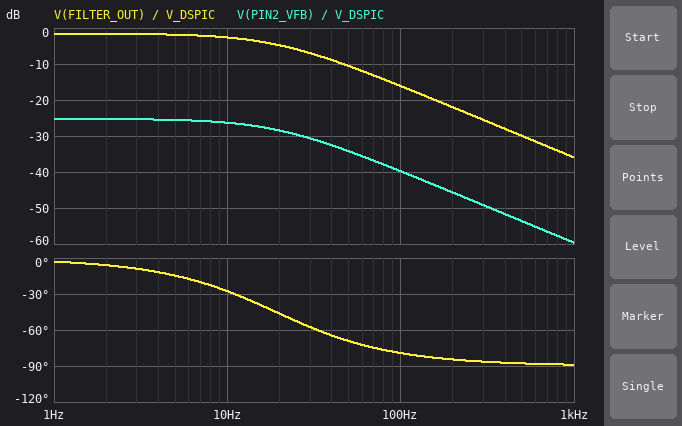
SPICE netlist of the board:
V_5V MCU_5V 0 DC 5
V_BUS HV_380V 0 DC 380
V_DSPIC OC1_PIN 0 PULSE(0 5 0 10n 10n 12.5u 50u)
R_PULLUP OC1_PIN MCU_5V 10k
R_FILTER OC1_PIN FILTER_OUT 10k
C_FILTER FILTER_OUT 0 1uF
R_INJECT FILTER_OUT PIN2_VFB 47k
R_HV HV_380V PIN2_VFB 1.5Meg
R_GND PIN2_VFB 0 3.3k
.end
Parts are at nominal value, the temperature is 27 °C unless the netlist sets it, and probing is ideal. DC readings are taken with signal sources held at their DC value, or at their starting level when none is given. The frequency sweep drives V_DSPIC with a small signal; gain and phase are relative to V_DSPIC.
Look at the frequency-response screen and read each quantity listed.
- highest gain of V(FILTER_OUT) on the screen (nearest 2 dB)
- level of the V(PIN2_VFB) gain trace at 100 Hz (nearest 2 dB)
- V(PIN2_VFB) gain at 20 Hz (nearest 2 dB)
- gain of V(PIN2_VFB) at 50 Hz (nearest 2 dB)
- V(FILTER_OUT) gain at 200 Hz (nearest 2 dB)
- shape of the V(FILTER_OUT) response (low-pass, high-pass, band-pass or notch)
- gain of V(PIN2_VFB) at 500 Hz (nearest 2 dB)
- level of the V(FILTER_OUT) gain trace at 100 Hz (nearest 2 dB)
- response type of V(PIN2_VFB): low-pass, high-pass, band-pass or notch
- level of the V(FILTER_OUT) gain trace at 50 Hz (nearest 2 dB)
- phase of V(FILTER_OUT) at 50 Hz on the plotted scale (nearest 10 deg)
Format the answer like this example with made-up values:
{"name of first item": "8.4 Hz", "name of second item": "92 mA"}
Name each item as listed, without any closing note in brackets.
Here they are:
{"highest gain of V(FILTER_OUT) on the screen": "-2 dB", "level of the V(PIN2_VFB) gain trace at 100 Hz": "-40 dB", "V(PIN2_VFB) gain at 20 Hz": "-28 dB", "gain of V(PIN2_VFB) at 50 Hz": "-34 dB", "V(FILTER_OUT) gain at 200 Hz": "-22 dB", "shape of the V(FILTER_OUT) response": "low-pass", "gain of V(PIN2_VFB) at 500 Hz": "-54 dB", "level of the V(FILTER_OUT) gain trace at 100 Hz": "-16 dB", "response type of V(PIN2_VFB): low-pass, high-pass, band-pass or notch": "low-pass", "level of the V(FILTER_OUT) gain trace at 50 Hz": "-10 dB", "phase of V(FILTER_OUT) at 50 Hz on the plotted scale": "-70 deg"}
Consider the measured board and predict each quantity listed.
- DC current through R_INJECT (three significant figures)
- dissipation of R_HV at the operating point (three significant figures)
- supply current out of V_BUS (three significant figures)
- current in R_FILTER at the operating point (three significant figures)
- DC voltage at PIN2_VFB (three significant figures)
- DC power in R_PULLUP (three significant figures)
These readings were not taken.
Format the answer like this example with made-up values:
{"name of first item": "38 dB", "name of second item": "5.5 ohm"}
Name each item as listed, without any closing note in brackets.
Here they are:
{"DC current through R_INJECT": "13.8 µA", "dissipation of R_HV at the operating point": "95.9 mW", "supply current out of V_BUS": "253 µA", "current in R_FILTER at the operating point": "13.8 µA", "DC voltage at PIN2_VFB": "789 mV", "DC power in R_PULLUP": "2.50 mW"}
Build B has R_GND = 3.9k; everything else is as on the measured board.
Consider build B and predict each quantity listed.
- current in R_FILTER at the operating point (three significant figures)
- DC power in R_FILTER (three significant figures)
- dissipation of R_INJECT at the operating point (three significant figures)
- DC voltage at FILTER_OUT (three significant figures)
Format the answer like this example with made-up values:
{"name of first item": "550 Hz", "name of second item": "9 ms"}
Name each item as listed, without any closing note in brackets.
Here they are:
{"current in R_FILTER at the operating point": "16.2 µA", "DC power in R_FILTER": "2.62 µW", "dissipation of R_INJECT at the operating point": "12.3 µW", "DC voltage at FILTER_OUT": "162 mV"}
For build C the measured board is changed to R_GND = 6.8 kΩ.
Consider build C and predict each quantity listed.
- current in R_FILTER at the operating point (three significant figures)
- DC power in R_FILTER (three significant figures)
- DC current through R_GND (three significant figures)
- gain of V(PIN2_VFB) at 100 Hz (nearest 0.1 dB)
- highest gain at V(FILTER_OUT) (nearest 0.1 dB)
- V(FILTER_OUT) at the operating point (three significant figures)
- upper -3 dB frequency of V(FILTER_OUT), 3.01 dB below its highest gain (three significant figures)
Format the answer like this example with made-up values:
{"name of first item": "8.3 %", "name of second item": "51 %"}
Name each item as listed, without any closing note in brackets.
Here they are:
{"current in R_FILTER at the operating point": "26.9 µA", "DC power in R_FILTER": "7.23 µW", "DC current through R_GND": "225 µA", "gain of V(PIN2_VFB) at 100 Hz": "-34.1 dB", "highest gain at V(FILTER_OUT)": "-1.5 dB", "V(FILTER_OUT) at the operating point": "269 mV", "upper -3 dB frequency of V(FILTER_OUT), 3.01 dB below its highest gain": "18.9 Hz"}
